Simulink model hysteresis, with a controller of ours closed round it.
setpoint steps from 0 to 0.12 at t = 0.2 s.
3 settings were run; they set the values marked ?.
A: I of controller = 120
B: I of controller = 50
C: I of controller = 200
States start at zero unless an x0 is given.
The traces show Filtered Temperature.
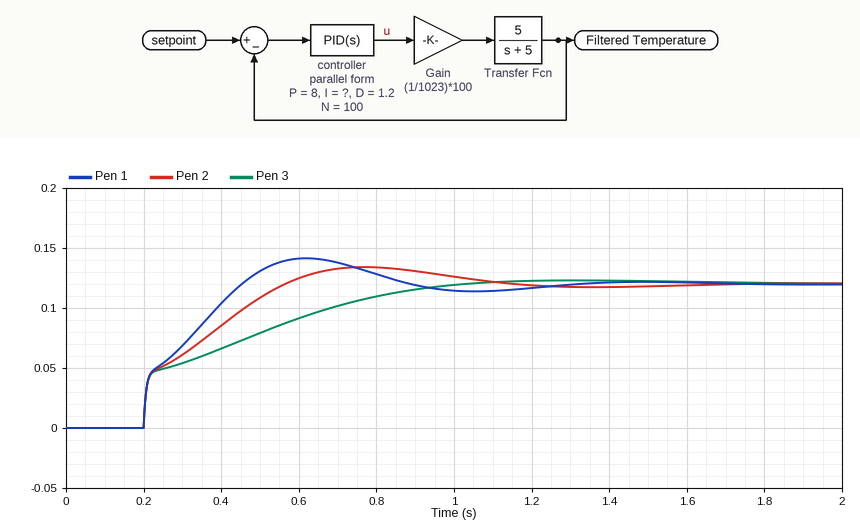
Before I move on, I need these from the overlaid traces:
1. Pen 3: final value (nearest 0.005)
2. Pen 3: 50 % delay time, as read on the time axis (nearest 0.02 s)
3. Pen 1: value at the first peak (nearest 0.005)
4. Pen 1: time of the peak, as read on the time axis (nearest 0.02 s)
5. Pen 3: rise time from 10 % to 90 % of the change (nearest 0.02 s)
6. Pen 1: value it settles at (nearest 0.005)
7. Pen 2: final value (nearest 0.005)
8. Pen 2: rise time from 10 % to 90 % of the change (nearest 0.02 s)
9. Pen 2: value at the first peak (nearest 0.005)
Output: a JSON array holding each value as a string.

["0.120", "0.36 s", "0.140", "0.62 s", "0.58 s", "0.120", "0.120", "0.30 s", "0.135"]
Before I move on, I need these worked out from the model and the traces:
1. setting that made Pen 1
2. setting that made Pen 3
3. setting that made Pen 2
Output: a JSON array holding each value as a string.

["C", "B", "A"]
